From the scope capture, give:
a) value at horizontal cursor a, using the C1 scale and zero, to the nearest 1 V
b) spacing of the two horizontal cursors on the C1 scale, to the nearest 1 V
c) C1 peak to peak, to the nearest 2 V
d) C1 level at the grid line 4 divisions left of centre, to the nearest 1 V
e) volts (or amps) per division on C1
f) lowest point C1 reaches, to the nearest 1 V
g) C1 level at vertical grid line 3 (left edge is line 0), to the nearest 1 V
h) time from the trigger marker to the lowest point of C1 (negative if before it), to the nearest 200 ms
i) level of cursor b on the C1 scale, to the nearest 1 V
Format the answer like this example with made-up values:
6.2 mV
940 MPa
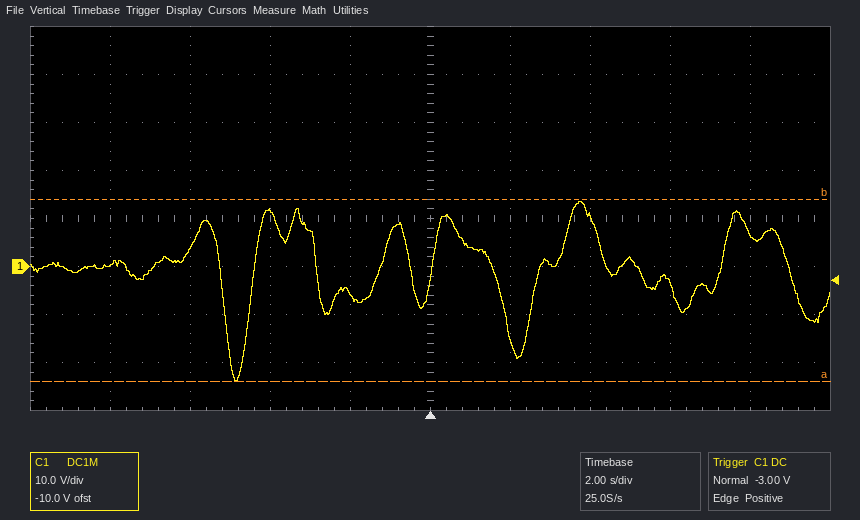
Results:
-24 V
38 V
38 V
1 V
10 V
-24 V
11 V
-4.8 s
14 V
